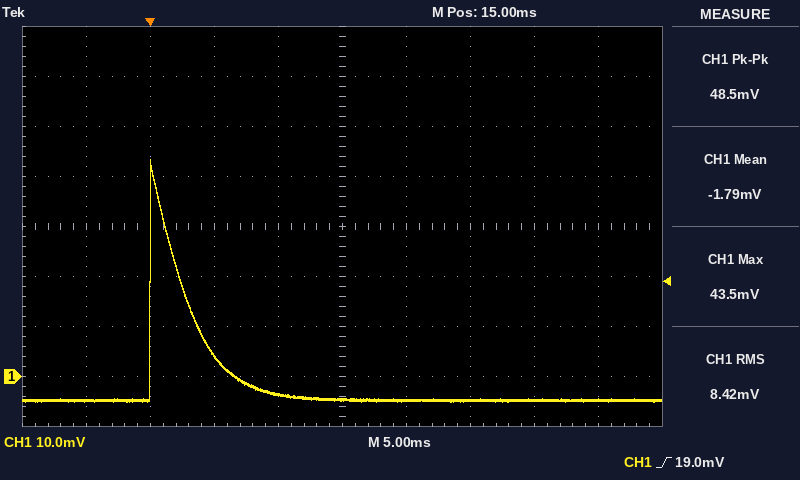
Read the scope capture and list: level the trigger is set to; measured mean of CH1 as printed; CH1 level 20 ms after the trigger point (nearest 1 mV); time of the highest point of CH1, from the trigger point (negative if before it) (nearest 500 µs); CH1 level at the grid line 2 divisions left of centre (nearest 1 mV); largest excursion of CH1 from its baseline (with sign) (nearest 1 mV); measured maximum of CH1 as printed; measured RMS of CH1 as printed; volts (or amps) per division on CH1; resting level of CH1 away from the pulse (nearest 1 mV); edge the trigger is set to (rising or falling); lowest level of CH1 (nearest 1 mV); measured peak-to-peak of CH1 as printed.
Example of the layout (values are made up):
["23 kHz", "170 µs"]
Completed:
["19.0 mV", "-1.79 mV", "-5 mV", "0.0 ms", "4 mV", "+48 mV", "43.5 mV", "8.42 mV", "10 mV", "-5 mV", "rising", "-5 mV", "48.5 mV"]
